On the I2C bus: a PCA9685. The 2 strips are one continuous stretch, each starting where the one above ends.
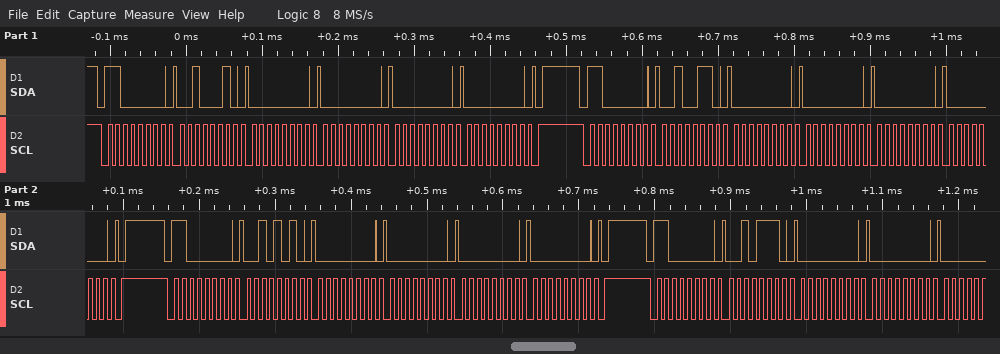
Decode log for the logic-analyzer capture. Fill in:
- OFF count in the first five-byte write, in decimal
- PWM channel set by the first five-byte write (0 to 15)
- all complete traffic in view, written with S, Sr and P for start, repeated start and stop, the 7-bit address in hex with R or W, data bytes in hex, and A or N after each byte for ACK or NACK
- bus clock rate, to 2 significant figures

0
7
S 60W A 22 A 00 A 00 A 00 A 00 A P S 60W A 26 A 00 A 00 A 00 A 00 A P S 60W A 2A A 00 A 00 A 00 A 00 A P S 60W A 2E A 00 A 00 A
100 kHz
